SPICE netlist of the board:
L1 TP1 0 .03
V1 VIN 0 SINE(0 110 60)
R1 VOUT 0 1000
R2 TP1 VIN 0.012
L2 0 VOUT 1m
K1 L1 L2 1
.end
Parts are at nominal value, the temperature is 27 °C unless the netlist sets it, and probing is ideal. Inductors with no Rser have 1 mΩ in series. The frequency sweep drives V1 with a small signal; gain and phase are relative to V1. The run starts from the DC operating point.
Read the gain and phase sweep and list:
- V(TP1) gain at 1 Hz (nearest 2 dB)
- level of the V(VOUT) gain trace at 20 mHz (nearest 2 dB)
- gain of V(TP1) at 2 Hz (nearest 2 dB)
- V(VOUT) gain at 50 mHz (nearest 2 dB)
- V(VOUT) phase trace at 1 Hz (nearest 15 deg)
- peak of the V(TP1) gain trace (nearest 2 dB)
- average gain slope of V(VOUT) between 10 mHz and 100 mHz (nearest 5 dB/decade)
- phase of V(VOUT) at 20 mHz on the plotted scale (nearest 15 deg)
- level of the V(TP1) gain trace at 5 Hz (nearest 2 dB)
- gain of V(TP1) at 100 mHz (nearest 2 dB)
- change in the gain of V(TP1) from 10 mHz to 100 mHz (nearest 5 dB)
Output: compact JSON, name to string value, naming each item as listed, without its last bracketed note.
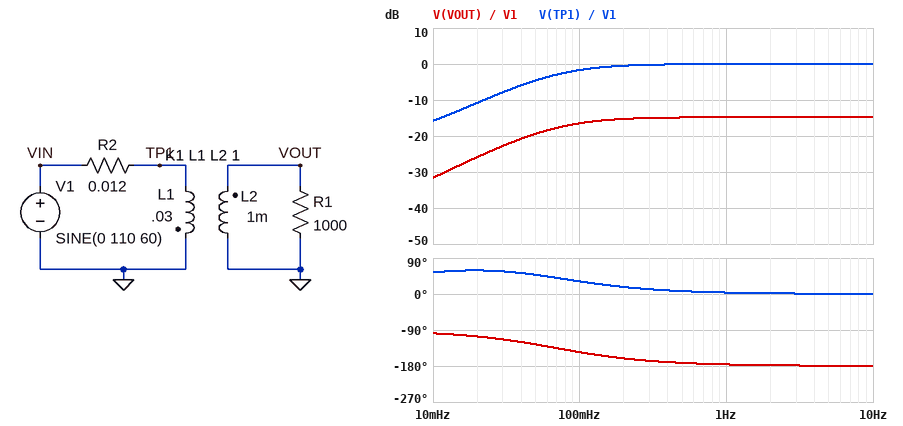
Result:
{"V(TP1) gain at 1 Hz": "0 dB", "level of the V(VOUT) gain trace at 20 mHz": "-26 dB", "gain of V(TP1) at 2 Hz": "0 dB", "V(VOUT) gain at 50 mHz": "-20 dB", "V(VOUT) phase trace at 1 Hz": "-180 deg", "peak of the V(TP1) gain trace": "0 dB", "average gain slope of V(VOUT) between 10 mHz and 100 mHz": "15 dB/decade", "phase of V(VOUT) at 20 mHz on the plotted scale": "-105 deg", "level of the V(TP1) gain trace at 5 Hz": "0 dB", "gain of V(TP1) at 100 mHz": "-2 dB", "change in the gain of V(TP1) from 10 mHz to 100 mHz": "15 dB"}
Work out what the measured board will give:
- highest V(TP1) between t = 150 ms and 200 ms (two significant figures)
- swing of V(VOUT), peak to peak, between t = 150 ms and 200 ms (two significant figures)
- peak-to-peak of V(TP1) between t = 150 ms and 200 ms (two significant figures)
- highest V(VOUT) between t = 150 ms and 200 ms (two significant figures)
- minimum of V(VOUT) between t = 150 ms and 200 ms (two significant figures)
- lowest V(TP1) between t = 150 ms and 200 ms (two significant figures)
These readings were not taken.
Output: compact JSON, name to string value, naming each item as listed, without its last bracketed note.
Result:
{"highest V(TP1) between t = 150 ms and 200 ms": "110 V", "swing of V(VOUT), peak to peak, between t = 150 ms and 200 ms": "40 V", "peak-to-peak of V(TP1) between t = 150 ms and 200 ms": "220 V", "highest V(VOUT) between t = 150 ms and 200 ms": "20 V", "minimum of V(VOUT) between t = 150 ms and 200 ms": "-20 V", "lowest V(TP1) between t = 150 ms and 200 ms": "-110 V"}
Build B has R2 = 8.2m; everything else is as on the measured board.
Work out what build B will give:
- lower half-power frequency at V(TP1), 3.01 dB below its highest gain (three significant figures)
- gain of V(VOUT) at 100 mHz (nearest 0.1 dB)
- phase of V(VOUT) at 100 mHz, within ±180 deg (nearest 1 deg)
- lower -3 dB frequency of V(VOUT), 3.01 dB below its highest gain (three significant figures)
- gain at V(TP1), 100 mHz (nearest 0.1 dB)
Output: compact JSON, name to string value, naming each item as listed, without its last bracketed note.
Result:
{"lower half-power frequency at V(TP1), 3.01 dB below its highest gain": "48.2 mHz", "gain of V(VOUT) at 100 mHz": "-15.7 dB", "phase of V(VOUT) at 100 mHz, within ±180 deg": "-154 deg", "lower -3 dB frequency of V(VOUT), 3.01 dB below its highest gain": "48.8 mHz", "gain at V(TP1), 100 mHz": "-0.9 dB"}
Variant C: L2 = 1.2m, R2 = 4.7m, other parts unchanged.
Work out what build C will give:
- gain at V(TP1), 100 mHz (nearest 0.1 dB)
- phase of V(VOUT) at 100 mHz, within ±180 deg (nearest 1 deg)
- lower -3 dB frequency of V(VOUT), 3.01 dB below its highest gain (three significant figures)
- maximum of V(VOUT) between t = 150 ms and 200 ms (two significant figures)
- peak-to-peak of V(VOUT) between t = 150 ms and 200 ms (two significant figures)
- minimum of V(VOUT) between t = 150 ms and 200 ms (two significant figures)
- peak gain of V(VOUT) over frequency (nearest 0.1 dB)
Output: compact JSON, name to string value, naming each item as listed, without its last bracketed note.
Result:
{"gain at V(TP1), 100 mHz": "-0.4 dB", "phase of V(VOUT) at 100 mHz, within ±180 deg": "-163 deg", "lower -3 dB frequency of V(VOUT), 3.01 dB below its highest gain": "30.2 mHz", "maximum of V(VOUT) between t = 150 ms and 200 ms": "22 V", "peak-to-peak of V(VOUT) between t = 150 ms and 200 ms": "44 V", "minimum of V(VOUT) between t = 150 ms and 200 ms": "-22 V", "peak gain of V(VOUT) over frequency": "-14.0 dB"}
